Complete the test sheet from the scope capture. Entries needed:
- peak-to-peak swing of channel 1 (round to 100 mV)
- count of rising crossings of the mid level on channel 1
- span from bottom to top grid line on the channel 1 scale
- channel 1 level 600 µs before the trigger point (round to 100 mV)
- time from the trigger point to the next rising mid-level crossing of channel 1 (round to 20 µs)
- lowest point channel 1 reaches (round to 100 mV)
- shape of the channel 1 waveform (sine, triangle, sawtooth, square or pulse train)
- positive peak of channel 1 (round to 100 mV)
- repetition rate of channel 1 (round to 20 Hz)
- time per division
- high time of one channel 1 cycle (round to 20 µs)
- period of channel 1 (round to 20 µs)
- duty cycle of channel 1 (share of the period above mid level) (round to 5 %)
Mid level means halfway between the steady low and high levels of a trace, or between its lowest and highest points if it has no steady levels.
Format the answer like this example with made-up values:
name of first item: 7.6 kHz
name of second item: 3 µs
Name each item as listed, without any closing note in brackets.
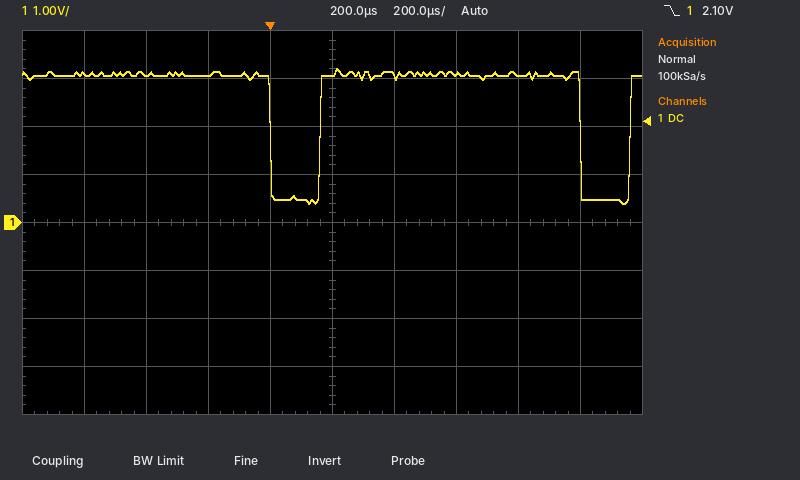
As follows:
peak-to-peak swing of channel 1: 2.8 V
count of rising crossings of the mid level on channel 1: 2
span from bottom to top grid line on the channel 1 scale: 8 V
channel 1 level 600 µs before the trigger point: 3.1 V
time from the trigger point to the next rising mid-level crossing of channel 1: 160 µs
lowest point channel 1 reaches: 400 mV
shape of the channel 1 waveform: pulse train
positive peak of channel 1: 3.2 V
repetition rate of channel 1: 1.00 kHz
time per division: 200 µs
high time of one channel 1 cycle: 840 µs
period of channel 1: 1.00 ms
duty cycle of channel 1 (share of the period above mid level): 85 %
